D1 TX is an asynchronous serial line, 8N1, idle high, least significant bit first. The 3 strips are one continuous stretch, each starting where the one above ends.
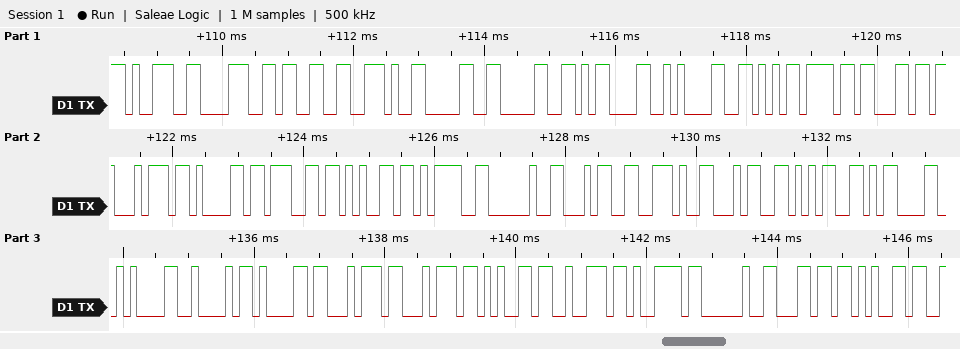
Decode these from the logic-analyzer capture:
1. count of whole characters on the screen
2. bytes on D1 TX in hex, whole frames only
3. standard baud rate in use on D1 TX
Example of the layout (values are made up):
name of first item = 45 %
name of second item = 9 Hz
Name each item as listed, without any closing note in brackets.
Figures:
count of whole characters on the screen = 33
bytes on D1 TX in hex, whole frames only = 39 38 33 2E 30 30 0D 0A 56 6F 6C 74 61 67 65 3D 20 34 2E 34 35 0D 0A 42 61 74 74 65 72 79 20 6C 65
standard baud rate in use on D1 TX = 9600 baud
